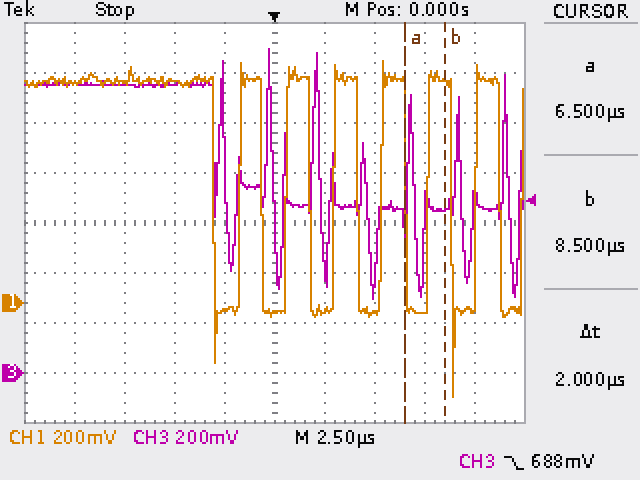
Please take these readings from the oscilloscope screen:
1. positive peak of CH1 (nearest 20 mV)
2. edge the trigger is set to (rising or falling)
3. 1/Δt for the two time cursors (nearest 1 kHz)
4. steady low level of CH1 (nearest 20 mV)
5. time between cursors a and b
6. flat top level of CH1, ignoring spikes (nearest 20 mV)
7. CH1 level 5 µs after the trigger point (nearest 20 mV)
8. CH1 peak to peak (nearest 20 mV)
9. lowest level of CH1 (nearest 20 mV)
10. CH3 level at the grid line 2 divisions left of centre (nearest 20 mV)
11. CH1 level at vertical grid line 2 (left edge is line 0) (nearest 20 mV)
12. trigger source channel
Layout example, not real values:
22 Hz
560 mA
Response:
960 mV
falling
500 kHz
-40 mV
2 µs
880 mV
-40 mV
1.34 V
-380 mV
1.16 V
880 mV
CH3
